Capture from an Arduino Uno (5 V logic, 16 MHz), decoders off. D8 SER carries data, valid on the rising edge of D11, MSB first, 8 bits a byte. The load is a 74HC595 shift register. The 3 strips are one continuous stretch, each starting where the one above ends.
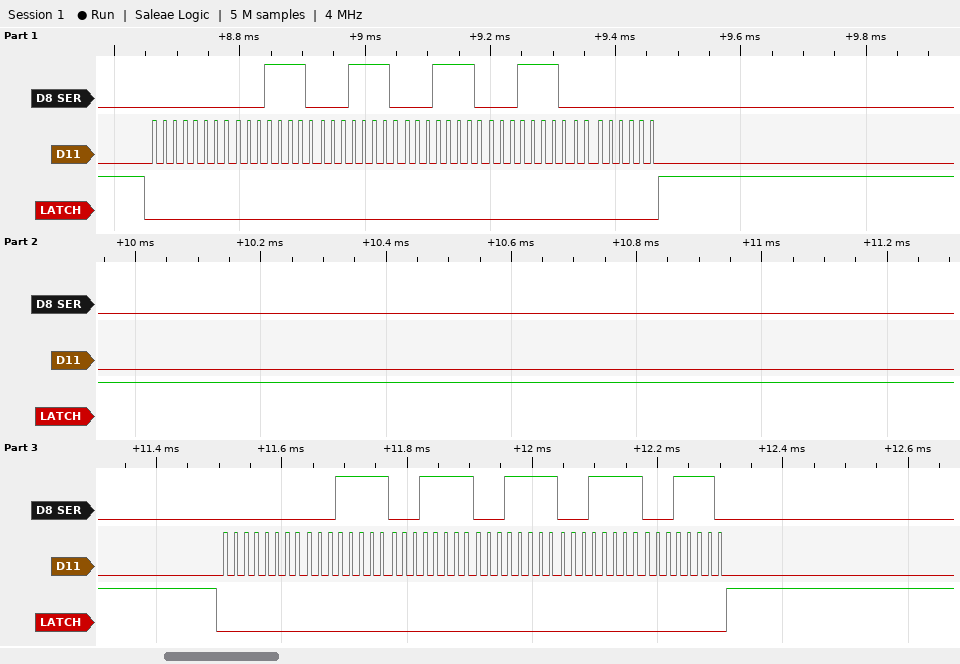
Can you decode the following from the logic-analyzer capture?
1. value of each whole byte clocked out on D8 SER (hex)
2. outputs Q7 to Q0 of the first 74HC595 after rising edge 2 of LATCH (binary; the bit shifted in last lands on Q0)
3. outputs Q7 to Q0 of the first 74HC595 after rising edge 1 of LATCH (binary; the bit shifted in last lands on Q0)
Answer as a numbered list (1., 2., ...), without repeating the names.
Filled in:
1. 00 1E 1E 1E 1E 00 00 1F 1F 1F 1F 1E
2. 00011110
3. 00000000
